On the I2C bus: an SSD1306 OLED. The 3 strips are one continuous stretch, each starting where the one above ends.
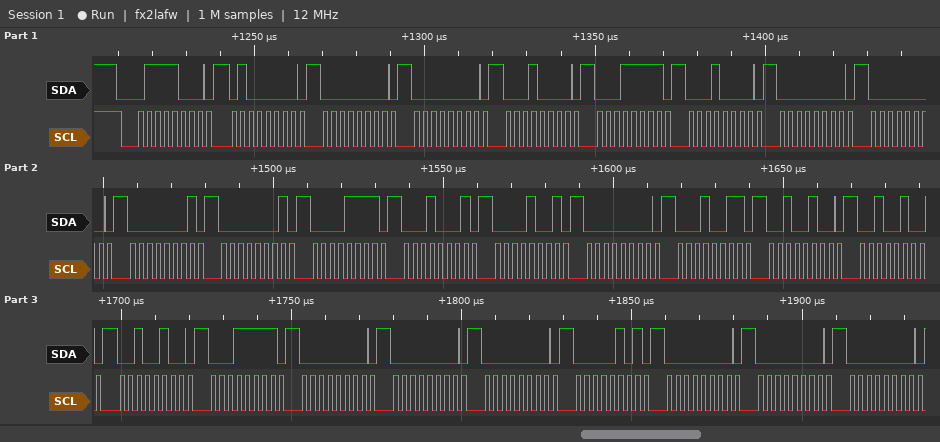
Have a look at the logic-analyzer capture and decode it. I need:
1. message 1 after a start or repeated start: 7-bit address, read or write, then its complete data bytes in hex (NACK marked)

0x3C write: 40 00 00 10 1F 10 00 00 01 01 0F 11 09 00 13 24 24 24 1F 00 00 00 05 00 00 00
